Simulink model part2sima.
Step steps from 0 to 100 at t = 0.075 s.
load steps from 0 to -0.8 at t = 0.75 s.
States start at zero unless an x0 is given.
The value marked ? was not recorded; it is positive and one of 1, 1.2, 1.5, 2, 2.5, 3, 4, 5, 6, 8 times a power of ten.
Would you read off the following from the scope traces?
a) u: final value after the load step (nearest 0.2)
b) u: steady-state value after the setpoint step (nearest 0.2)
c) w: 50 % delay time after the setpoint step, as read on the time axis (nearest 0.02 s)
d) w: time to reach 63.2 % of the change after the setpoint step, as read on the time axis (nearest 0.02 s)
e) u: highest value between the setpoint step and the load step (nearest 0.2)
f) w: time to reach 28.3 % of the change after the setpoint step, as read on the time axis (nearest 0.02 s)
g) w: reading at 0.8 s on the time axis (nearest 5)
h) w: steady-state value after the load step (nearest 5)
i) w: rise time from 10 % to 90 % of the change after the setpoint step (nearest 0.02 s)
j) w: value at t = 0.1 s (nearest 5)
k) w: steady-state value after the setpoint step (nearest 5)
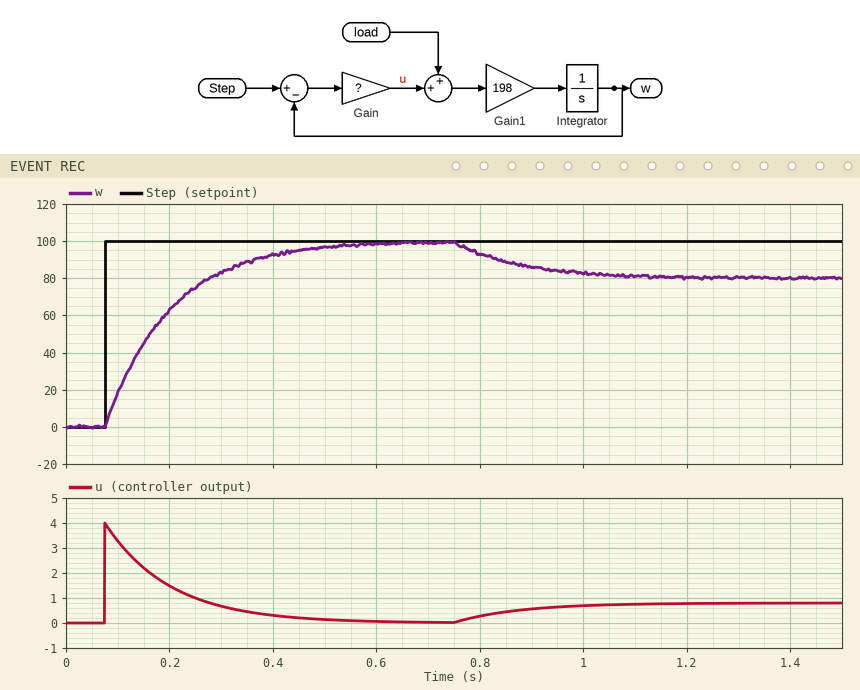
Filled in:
0.8
0.0
0.16 s
0.20 s
4.0
0.12 s
95
80
0.28 s
20
100
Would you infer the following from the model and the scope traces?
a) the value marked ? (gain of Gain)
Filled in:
0.04
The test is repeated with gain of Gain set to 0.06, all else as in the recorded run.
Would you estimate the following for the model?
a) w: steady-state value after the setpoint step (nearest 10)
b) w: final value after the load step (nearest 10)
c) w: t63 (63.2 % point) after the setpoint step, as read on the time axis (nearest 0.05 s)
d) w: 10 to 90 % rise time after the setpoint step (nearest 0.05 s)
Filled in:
100
90
0.15 s
0.20 s
